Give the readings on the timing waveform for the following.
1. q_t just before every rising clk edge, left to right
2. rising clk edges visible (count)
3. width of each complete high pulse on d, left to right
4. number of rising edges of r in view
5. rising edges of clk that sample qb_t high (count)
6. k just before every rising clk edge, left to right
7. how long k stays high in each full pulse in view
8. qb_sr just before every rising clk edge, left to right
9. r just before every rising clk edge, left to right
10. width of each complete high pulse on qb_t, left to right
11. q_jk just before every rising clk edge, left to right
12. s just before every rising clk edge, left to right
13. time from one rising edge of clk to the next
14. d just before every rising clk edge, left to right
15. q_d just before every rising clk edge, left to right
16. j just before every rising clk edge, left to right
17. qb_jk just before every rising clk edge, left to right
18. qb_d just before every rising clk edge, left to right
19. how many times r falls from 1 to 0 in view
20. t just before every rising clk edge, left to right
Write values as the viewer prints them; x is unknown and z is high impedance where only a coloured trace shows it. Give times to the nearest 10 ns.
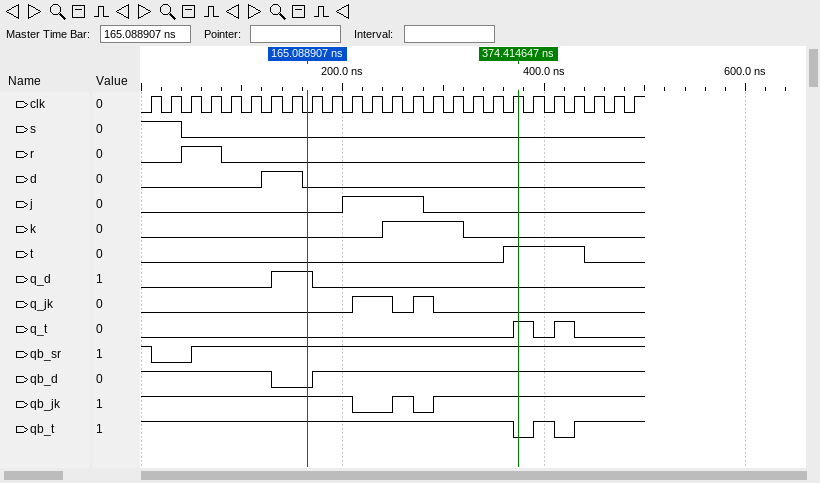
0 0 0 0 0 0 0 0 0 0 0 0 0 0 0 0 0 0 0 1 0 1 0 0 0
25
40 ns
1
23
0 0 0 0 0 0 0 0 0 0 0 0 1 1 1 1 0 0 0 0 0 0 0 0 0
80 ns
1 0 0 1 1 1 1 1 1 1 1 1 1 1 1 1 1 1 1 1 1 1 1 1 1
0 0 1 1 0 0 0 0 0 0 0 0 0 0 0 0 0 0 0 0 0 0 0 0 0
20 ns
0 0 0 0 0 0 0 0 0 0 0 1 1 0 1 0 0 0 0 0 0 0 0 0 0
1 1 0 0 0 0 0 0 0 0 0 0 0 0 0 0 0 0 0 0 0 0 0 0 0
20 ns
0 0 0 0 0 0 1 1 0 0 0 0 0 0 0 0 0 0 0 0 0 0 0 0 0
0 0 0 0 0 0 0 1 1 0 0 0 0 0 0 0 0 0 0 0 0 0 0 0 0
0 0 0 0 0 0 0 0 0 0 1 1 1 1 0 0 0 0 0 0 0 0 0 0 0
1 1 1 1 1 1 1 1 1 1 1 0 0 1 0 1 1 1 1 1 1 1 1 1 1
1 1 1 1 1 1 1 0 0 1 1 1 1 1 1 1 1 1 1 1 1 1 1 1 1
1
0 0 0 0 0 0 0 0 0 0 0 0 0 0 0 0 0 0 1 1 1 1 0 0 0
